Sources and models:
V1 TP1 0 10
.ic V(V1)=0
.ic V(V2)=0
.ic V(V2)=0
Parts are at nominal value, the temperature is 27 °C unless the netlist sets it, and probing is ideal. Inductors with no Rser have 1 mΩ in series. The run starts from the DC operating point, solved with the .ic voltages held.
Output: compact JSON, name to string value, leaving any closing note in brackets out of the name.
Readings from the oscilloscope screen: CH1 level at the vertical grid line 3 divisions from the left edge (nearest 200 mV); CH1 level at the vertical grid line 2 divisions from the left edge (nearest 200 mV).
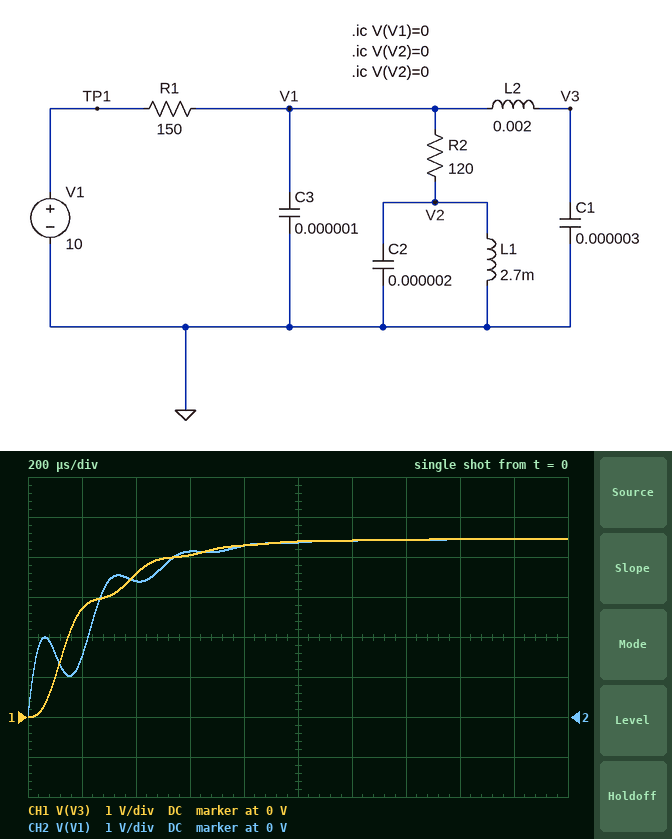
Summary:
{"CH1 level at the vertical grid line 3 divisions from the left edge": "4.0 V", "CH1 level at the vertical grid line 2 divisions from the left edge": "3.6 V"}
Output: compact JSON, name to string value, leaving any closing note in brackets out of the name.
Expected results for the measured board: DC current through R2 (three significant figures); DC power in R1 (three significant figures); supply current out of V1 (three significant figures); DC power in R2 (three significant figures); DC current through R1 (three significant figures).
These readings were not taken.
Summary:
{"DC current through R2": "37.0 mA", "DC power in R1": "206 mW", "supply current out of V1": "37.0 mA", "DC power in R2": "165 mW", "DC current through R1": "37.0 mA"}
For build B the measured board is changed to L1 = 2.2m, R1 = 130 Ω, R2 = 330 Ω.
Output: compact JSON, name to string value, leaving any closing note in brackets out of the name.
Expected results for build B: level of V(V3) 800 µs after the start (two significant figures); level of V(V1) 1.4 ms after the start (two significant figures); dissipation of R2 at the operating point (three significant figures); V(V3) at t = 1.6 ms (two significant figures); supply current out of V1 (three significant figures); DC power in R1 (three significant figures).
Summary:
{"level of V(V3) 800 µs after the start": "6.4 V", "level of V(V1) 1.4 ms after the start": "7.0 V", "dissipation of R2 at the operating point": "156 mW", "V(V3) at t = 1.6 ms": "7.1 V", "supply current out of V1": "21.7 mA", "DC power in R1": "61.4 mW"}
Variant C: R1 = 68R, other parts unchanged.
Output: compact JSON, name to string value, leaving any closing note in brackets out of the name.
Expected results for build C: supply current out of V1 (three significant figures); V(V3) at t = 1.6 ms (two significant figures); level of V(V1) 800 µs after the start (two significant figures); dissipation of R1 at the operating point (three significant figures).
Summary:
{"supply current out of V1": "53.2 mA", "V(V3) at t = 1.6 ms": "6.4 V", "level of V(V1) 800 µs after the start": "6.3 V", "dissipation of R1 at the operating point": "192 mW"}
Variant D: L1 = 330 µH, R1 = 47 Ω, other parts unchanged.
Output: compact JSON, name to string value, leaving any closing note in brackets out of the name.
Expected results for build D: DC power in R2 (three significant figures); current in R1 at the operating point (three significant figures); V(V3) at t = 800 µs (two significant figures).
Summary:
{"DC power in R2": "430 mW", "current in R1 at the operating point": "59.9 mA", "V(V3) at t = 800 µs": "7.2 V"}
